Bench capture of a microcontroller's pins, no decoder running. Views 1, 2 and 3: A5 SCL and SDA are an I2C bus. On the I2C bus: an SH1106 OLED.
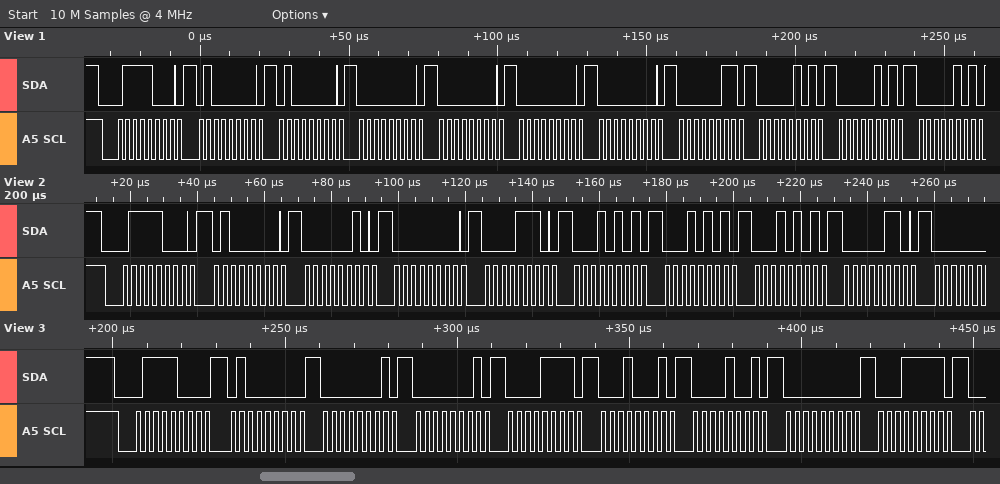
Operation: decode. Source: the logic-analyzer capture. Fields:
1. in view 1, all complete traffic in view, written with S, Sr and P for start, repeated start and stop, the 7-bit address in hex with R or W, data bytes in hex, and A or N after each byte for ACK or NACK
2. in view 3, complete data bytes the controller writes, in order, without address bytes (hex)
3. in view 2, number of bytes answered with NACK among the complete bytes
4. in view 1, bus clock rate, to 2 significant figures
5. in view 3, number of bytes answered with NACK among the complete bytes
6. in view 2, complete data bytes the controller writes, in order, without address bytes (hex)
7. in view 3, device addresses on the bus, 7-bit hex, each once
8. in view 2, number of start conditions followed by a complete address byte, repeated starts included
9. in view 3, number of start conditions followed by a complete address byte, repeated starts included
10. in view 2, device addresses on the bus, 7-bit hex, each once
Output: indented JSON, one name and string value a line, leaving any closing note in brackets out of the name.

{
  "in view 1, all complete traffic in view, written with S, Sr and P for start, repeated start and stop, the 7-bit address in hex with R or W, data bytes in hex, and A or N after each byte for ACK or NACK": "S 3CW A 40 A 40 A 00 A 00 A 00 A 00 A 03 A 05 A 05 A 05 A",
  "in view 3, complete data bytes the controller writes, in order, without address bytes": "40 01 01 0F 11 09 00 1F",
  "in view 2, number of bytes answered with NACK among the complete bytes": "0",
  "in view 1, bus clock rate, to 2 significant figures": "400 kHz",
  "in view 3, number of bytes answered with NACK among the complete bytes": "0",
  "in view 2, complete data bytes the controller writes, in order, without address bytes": "40 02 00 0E 15 15 15 06",
  "in view 3, device addresses on the bus, 7-bit hex, each once": "0x3C",
  "in view 2, number of start conditions followed by a complete address byte, repeated starts included": "1",
  "in view 3, number of start conditions followed by a complete address byte, repeated starts included": "1",
  "in view 2, device addresses on the bus, 7-bit hex, each once": "0x3C"
}
